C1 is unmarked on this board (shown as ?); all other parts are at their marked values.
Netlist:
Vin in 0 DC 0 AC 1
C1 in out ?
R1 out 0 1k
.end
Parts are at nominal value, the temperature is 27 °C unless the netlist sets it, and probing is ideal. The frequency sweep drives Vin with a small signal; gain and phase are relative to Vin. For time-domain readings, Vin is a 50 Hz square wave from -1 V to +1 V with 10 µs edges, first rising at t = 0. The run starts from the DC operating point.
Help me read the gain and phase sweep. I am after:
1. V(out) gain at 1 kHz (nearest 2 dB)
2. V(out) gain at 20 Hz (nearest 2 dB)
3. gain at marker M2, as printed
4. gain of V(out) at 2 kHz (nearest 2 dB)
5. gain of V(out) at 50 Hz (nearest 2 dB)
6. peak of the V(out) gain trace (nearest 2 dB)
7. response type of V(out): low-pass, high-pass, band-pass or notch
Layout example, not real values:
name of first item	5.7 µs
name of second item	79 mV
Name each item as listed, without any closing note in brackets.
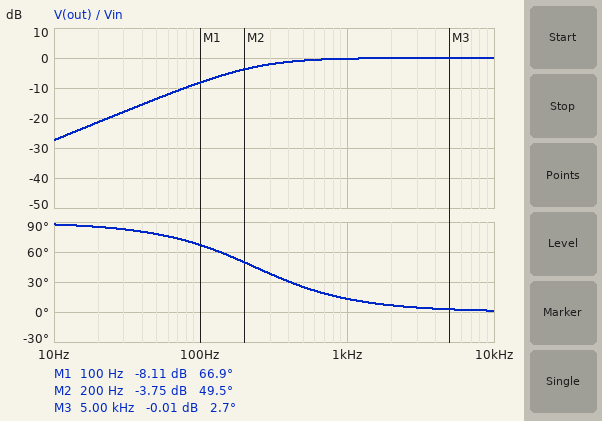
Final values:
V(out) gain at 1 kHz	0 dB
V(out) gain at 20 Hz	-22 dB
gain at marker M2, as printed	-3.75 dB
gain of V(out) at 2 kHz	0 dB
gain of V(out) at 50 Hz	-14 dB
peak of the V(out) gain trace	0 dB
response type of V(out): low-pass, high-pass, band-pass or notch	high-pass
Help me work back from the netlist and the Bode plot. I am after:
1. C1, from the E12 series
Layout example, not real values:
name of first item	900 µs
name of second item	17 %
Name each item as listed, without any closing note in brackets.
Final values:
C1, from the E12 series	680 nF
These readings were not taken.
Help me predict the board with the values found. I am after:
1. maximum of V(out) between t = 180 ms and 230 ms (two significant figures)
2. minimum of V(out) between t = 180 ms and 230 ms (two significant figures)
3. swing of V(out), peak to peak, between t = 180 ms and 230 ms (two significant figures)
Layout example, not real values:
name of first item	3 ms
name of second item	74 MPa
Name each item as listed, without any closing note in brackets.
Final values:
maximum of V(out) between t = 180 ms and 230 ms	2.0 V
minimum of V(out) between t = 180 ms and 230 ms	-2.0 V
swing of V(out), peak to peak, between t = 180 ms and 230 ms	4.0 V
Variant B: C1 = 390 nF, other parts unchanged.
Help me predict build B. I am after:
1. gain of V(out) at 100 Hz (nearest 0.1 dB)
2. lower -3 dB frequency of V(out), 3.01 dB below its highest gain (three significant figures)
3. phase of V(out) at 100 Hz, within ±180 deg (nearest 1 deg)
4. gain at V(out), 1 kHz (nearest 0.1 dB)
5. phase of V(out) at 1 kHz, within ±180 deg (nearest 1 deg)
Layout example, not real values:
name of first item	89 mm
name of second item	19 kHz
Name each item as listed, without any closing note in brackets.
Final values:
gain of V(out) at 100 Hz	-12.5 dB
lower -3 dB frequency of V(out), 3.01 dB below its highest gain	408 Hz
phase of V(out) at 100 Hz, within ±180 deg	76 deg
gain at V(out), 1 kHz	-0.7 dB
phase of V(out) at 1 kHz, within ±180 deg	22 deg
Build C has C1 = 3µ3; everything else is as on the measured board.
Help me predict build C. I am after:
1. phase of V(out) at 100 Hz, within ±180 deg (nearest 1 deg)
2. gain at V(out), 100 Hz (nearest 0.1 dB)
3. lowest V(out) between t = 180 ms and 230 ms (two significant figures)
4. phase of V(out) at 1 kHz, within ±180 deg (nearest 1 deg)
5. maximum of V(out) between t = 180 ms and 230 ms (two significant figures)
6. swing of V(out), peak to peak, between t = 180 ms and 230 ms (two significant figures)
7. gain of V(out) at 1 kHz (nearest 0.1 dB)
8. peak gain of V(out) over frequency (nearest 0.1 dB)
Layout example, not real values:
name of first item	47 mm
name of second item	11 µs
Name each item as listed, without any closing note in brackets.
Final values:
phase of V(out) at 100 Hz, within ±180 deg	26 deg
gain at V(out), 100 Hz	-0.9 dB
lowest V(out) between t = 180 ms and 230 ms	-1.9 V
phase of V(out) at 1 kHz, within ±180 deg	3 deg
maximum of V(out) between t = 180 ms and 230 ms	1.9 V
swing of V(out), peak to peak, between t = 180 ms and 230 ms	3.8 V
gain of V(out) at 1 kHz	0 dB
peak gain of V(out) over frequency	0 dB
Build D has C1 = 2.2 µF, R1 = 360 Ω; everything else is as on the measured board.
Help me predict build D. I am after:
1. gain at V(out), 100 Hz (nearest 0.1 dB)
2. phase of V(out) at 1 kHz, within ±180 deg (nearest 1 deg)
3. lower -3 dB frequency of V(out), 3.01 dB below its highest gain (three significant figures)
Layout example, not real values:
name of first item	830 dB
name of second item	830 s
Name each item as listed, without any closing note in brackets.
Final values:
gain at V(out), 100 Hz	-7.0 dB
phase of V(out) at 1 kHz, within ±180 deg	11 deg
lower -3 dB frequency of V(out), 3.01 dB below its highest gain	201 Hz
